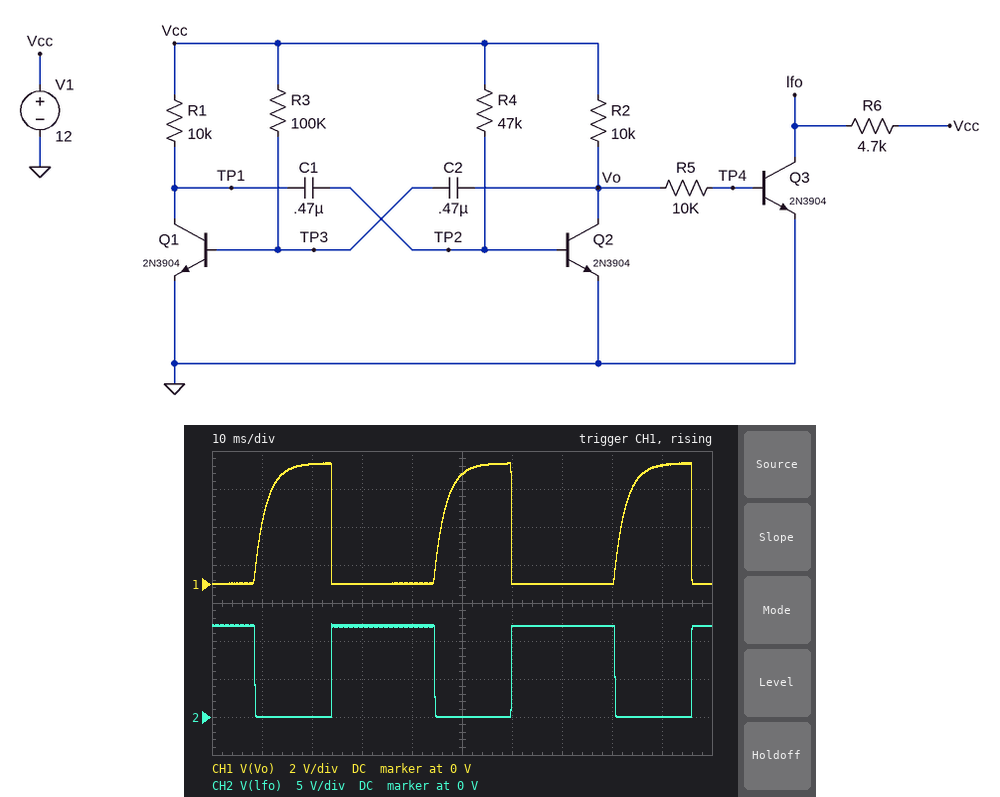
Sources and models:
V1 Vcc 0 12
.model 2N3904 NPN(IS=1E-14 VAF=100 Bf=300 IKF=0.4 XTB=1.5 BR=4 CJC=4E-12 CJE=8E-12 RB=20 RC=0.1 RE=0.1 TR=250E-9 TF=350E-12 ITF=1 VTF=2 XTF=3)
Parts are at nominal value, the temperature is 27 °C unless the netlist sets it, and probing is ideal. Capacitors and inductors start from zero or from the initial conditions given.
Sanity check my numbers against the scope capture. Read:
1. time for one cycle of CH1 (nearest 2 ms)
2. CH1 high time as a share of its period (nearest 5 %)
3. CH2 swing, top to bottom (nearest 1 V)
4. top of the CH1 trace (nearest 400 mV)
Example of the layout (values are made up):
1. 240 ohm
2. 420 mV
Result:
1. 36 ms
2. 40 %
3. 12 V
4. 6.4 V
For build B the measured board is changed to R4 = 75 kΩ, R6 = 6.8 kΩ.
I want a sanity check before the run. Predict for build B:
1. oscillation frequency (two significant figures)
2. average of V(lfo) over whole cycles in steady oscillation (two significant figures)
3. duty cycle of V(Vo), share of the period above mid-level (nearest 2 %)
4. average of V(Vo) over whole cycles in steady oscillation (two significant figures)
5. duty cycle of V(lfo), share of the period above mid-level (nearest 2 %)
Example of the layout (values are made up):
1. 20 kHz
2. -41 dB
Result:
1. 22 Hz
2. 5.5 V
3. 52 %
4. 3.2 V
5. 46 %
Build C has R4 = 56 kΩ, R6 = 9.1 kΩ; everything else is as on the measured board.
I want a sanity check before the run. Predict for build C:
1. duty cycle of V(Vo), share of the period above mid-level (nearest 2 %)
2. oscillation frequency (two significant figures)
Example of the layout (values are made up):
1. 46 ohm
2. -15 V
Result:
1. 44 %
2. 26 Hz
